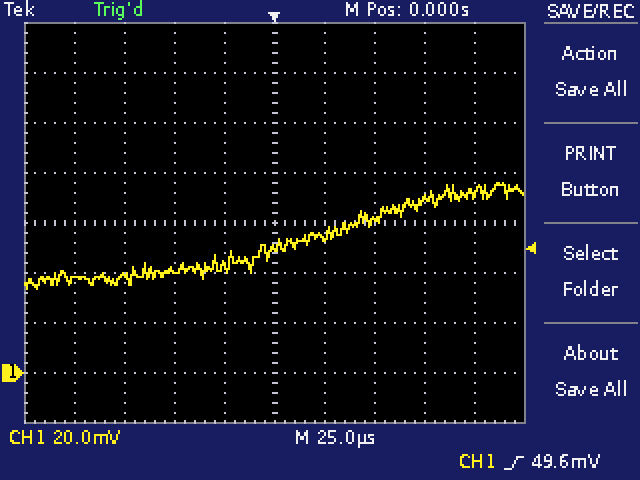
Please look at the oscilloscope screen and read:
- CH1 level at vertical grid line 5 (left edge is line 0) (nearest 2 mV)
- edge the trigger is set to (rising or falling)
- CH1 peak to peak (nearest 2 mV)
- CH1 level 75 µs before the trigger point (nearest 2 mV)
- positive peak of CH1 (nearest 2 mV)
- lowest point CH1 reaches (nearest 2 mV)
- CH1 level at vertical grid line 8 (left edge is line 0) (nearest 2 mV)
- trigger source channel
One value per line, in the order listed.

50 mV
rising
42 mV
38 mV
76 mV
34 mV
70 mV
CH1
